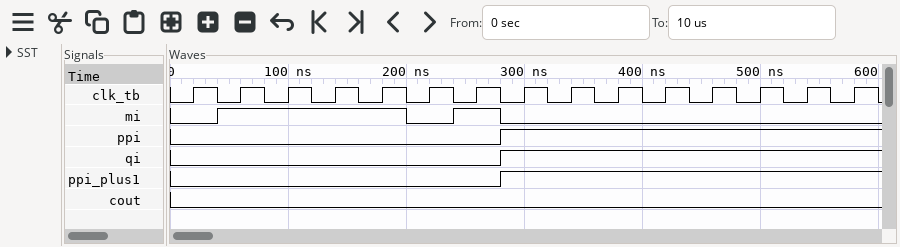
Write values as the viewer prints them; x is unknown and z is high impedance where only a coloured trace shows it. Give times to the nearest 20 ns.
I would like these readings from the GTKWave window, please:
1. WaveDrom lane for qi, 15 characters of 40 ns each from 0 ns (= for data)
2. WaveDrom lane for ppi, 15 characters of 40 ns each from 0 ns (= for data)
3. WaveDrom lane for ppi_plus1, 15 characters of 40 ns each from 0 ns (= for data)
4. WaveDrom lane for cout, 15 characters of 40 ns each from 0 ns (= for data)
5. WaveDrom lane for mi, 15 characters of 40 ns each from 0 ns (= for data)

{name: 'qi', wave: '0......1.......'}
{name: 'ppi', wave: '0......1.......'}
{name: 'ppi_plus1', wave: '0......1.......'}
{name: 'cout', wave: '0..............'}
{name: 'mi', wave: '01...010.......'}
